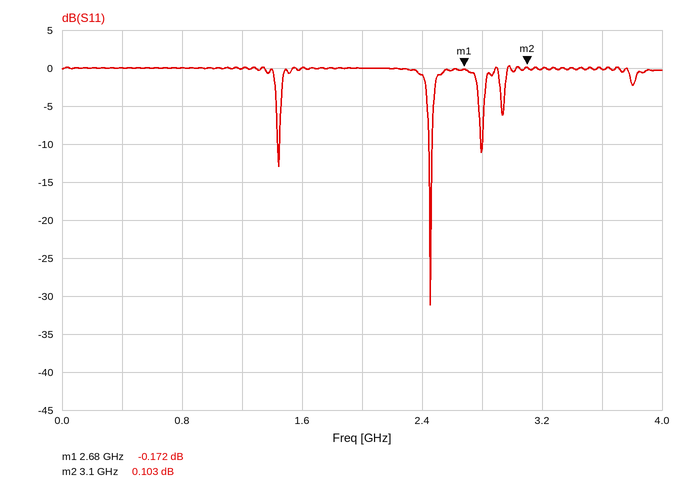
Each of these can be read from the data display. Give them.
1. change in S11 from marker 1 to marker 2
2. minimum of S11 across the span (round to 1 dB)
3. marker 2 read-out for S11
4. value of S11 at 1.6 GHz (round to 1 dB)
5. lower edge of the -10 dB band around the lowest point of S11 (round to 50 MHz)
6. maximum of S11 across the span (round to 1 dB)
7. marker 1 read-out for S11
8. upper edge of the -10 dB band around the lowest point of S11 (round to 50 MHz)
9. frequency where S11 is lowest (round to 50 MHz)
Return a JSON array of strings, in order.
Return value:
["0.275 dB", "-31 dB", "0.103 dB", "0 dB", "2.45 GHz", "0 dB", "-0.172 dB", "2.45 GHz", "2.45 GHz"]
